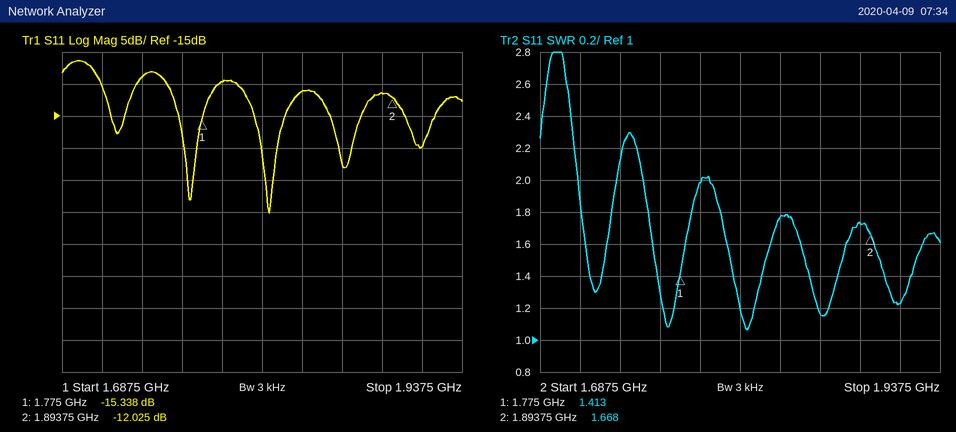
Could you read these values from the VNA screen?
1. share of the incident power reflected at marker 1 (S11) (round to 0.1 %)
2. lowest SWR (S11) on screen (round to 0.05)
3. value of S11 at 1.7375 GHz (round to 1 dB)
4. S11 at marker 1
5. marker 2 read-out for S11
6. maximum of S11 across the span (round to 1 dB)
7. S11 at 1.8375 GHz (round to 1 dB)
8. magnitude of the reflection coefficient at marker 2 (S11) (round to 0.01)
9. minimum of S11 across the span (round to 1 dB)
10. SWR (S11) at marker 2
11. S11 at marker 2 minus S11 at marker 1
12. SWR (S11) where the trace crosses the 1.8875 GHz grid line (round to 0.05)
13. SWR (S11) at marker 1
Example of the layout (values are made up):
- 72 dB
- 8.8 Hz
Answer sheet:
- 2.9 %
- 1.05
- -9 dB
- -15.338 dB
- -12.025 dB
- -6 dB
- -11 dB
- 0.25
- -30 dB
- 1.668
- 3.313 dB
- 1.75
- 1.413
